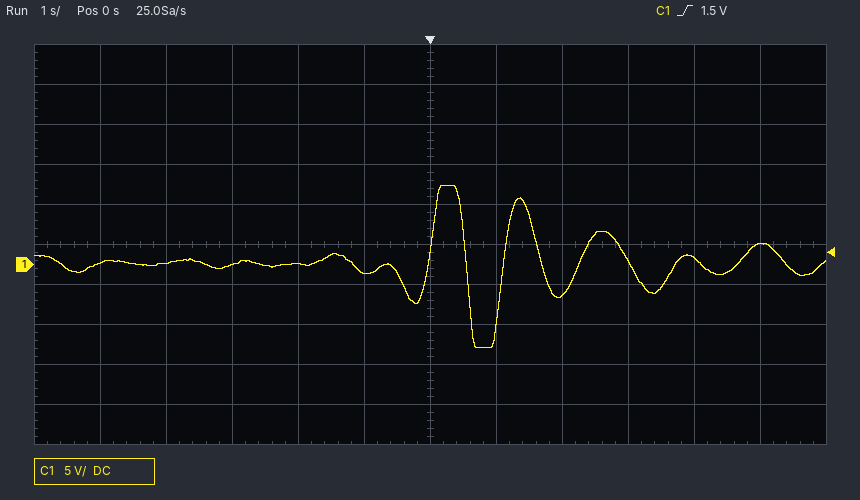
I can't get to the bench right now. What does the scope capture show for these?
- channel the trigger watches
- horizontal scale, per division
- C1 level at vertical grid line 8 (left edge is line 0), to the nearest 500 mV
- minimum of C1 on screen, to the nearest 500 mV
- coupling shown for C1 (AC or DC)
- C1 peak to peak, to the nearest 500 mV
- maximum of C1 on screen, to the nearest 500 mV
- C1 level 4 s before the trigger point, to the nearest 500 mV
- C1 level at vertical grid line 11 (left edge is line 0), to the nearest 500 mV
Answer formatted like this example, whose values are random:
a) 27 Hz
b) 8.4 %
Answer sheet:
a) C1
b) 1 s
c) -4.0 V
d) -10.5 V
e) DC
f) 20.5 V
g) 10.0 V
h) 0.0 V
i) 2.5 V
